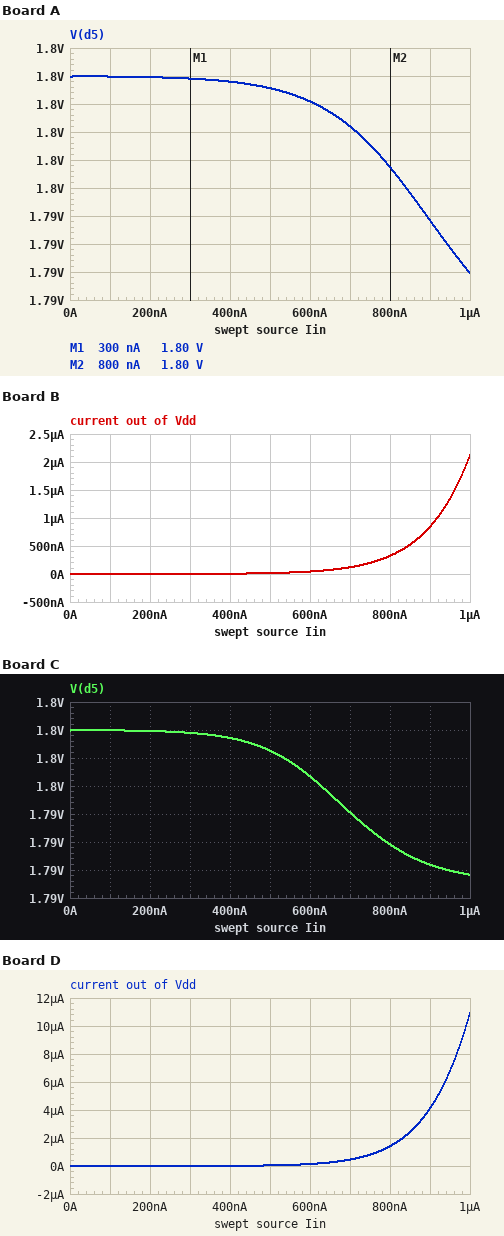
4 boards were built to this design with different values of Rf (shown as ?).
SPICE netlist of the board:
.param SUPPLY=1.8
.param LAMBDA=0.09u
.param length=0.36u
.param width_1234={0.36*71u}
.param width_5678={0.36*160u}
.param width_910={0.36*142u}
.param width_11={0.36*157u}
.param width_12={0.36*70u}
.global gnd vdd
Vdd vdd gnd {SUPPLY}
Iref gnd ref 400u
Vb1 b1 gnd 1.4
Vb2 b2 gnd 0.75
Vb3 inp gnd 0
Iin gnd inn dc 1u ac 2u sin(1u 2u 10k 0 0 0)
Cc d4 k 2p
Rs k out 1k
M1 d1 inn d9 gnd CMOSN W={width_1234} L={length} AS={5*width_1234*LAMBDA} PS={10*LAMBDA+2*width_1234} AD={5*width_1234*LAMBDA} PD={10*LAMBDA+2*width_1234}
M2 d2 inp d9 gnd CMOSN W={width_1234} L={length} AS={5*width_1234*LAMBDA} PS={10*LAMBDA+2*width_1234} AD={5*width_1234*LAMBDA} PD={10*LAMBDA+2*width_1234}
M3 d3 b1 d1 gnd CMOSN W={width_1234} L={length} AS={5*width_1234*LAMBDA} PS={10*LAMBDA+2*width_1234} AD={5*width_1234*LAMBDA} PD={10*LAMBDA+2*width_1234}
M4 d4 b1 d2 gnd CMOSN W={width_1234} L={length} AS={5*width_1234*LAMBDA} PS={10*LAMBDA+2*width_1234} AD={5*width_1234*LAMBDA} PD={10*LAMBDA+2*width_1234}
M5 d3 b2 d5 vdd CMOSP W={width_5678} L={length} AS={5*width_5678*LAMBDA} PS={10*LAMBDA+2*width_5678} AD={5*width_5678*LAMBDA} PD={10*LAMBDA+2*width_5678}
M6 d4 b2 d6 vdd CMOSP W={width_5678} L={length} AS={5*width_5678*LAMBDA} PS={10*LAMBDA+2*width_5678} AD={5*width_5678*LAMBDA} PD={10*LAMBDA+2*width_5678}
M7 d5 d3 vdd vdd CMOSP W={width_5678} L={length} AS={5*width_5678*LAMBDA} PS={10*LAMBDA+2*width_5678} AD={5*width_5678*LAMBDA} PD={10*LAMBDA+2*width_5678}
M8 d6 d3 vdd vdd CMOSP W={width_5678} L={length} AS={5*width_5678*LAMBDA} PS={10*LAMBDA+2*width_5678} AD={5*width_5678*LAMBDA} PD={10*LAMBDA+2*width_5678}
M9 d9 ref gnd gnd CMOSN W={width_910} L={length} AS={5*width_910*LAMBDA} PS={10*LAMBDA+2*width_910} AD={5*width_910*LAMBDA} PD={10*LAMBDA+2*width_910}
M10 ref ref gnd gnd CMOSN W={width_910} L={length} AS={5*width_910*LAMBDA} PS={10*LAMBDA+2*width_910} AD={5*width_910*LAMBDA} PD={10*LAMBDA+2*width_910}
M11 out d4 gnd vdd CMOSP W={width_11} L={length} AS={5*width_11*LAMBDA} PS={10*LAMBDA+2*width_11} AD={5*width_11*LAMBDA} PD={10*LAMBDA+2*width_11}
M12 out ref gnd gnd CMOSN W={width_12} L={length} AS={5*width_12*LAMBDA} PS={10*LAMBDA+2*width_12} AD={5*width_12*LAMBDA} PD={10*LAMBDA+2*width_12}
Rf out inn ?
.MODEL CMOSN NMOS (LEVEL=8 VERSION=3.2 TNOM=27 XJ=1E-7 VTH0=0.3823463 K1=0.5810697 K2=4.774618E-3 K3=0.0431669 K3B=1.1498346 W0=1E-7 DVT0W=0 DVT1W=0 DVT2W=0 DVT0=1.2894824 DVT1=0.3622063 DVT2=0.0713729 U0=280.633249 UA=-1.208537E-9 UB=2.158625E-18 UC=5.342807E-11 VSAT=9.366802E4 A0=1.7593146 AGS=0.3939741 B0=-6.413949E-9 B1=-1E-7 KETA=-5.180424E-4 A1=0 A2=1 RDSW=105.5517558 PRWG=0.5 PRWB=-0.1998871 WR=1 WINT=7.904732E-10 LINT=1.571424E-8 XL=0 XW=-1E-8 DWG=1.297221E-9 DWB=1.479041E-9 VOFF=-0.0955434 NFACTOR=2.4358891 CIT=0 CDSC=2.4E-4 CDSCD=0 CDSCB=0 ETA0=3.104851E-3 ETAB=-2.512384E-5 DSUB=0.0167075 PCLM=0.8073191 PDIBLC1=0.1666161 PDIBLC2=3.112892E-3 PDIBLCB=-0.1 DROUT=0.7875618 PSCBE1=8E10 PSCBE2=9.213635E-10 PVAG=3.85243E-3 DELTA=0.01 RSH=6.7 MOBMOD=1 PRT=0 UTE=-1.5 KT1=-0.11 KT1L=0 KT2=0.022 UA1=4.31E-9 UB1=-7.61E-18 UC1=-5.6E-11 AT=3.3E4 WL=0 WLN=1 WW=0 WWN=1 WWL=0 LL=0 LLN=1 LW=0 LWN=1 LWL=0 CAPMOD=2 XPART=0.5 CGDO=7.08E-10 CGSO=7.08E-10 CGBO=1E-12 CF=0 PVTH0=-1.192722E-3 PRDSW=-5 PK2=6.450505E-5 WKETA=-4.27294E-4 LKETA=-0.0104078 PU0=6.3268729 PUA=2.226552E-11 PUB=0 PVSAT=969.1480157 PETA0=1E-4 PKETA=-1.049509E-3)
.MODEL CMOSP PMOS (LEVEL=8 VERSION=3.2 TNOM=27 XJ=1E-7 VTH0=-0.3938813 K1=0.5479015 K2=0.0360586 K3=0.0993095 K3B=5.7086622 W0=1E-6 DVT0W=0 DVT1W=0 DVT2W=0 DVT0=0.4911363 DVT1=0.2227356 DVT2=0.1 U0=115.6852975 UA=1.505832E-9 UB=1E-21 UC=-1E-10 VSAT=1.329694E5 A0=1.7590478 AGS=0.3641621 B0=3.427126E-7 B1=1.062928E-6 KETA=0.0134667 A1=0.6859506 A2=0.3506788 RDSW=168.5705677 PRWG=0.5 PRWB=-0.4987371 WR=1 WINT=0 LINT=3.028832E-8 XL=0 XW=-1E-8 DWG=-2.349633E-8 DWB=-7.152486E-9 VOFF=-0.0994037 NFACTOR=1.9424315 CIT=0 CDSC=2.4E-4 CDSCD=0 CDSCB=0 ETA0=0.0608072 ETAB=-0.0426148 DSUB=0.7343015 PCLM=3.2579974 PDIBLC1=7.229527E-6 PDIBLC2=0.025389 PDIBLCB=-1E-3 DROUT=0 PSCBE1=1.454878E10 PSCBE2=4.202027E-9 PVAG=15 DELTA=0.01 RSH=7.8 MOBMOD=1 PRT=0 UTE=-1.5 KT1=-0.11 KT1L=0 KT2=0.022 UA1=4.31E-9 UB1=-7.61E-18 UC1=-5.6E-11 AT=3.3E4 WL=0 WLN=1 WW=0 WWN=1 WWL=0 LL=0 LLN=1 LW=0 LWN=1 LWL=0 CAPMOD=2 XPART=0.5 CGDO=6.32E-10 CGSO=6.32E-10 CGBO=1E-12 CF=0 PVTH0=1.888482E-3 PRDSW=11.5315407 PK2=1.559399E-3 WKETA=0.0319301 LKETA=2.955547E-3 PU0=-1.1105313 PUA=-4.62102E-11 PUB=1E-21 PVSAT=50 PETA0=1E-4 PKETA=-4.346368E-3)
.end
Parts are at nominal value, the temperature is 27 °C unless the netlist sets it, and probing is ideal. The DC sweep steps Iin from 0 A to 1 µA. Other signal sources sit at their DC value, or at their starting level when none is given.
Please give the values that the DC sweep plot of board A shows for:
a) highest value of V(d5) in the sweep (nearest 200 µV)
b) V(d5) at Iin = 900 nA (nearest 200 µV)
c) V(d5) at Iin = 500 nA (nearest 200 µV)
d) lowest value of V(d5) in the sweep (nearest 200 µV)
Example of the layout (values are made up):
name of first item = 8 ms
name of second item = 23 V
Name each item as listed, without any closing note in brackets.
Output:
highest value of V(d5) in the sweep = 1.8000 V
V(d5) at Iin = 900 nA = 1.7948 V
V(d5) at Iin = 500 nA = 1.7996 V
lowest value of V(d5) in the sweep = 1.7930 V
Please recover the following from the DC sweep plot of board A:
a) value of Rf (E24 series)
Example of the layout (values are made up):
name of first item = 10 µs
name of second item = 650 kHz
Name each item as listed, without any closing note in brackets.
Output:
value of Rf = 560 kΩ
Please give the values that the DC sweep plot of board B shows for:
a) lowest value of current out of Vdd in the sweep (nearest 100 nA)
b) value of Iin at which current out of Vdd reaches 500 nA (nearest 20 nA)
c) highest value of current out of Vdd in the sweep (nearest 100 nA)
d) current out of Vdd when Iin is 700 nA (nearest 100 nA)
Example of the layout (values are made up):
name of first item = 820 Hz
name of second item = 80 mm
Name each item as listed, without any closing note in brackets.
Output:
lowest value of current out of Vdd in the sweep = 0 A
value of Iin at which current out of Vdd reaches 500 nA = 840 nA
highest value of current out of Vdd in the sweep = 2.1 µA
current out of Vdd when Iin is 700 nA = 100 nA
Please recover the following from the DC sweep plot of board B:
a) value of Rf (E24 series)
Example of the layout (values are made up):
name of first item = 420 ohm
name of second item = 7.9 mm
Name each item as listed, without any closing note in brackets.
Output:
value of Rf = 360 kΩ
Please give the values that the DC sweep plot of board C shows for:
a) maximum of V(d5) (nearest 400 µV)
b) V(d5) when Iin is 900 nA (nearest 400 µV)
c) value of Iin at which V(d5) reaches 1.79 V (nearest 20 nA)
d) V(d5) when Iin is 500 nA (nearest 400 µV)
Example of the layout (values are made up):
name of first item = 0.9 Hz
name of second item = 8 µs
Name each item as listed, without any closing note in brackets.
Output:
maximum of V(d5) = 1.8000 V
V(d5) when Iin is 900 nA = 1.7904 V
value of Iin at which V(d5) reaches 1.79 V = 700 nA
V(d5) when Iin is 500 nA = 1.7984 V
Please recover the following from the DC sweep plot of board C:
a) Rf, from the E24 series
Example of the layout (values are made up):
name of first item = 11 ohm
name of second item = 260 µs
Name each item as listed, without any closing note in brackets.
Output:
Rf, from the E24 series = 750 kΩ
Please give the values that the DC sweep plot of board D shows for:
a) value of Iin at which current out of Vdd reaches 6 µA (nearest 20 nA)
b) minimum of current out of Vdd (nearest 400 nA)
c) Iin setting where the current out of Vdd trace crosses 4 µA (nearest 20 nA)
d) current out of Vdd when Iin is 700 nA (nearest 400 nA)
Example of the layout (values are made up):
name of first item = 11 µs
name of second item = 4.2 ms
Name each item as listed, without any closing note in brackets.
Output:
value of Iin at which current out of Vdd reaches 6 µA = 940 nA
minimum of current out of Vdd = 0 A
Iin setting where the current out of Vdd trace crosses 4 µA = 900 nA
current out of Vdd when Iin is 700 nA = 400 nA
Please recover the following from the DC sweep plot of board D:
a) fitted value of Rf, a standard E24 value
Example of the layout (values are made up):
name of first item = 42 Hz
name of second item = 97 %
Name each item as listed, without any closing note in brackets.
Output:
fitted value of Rf, a standard E24 value = 430 kΩ
